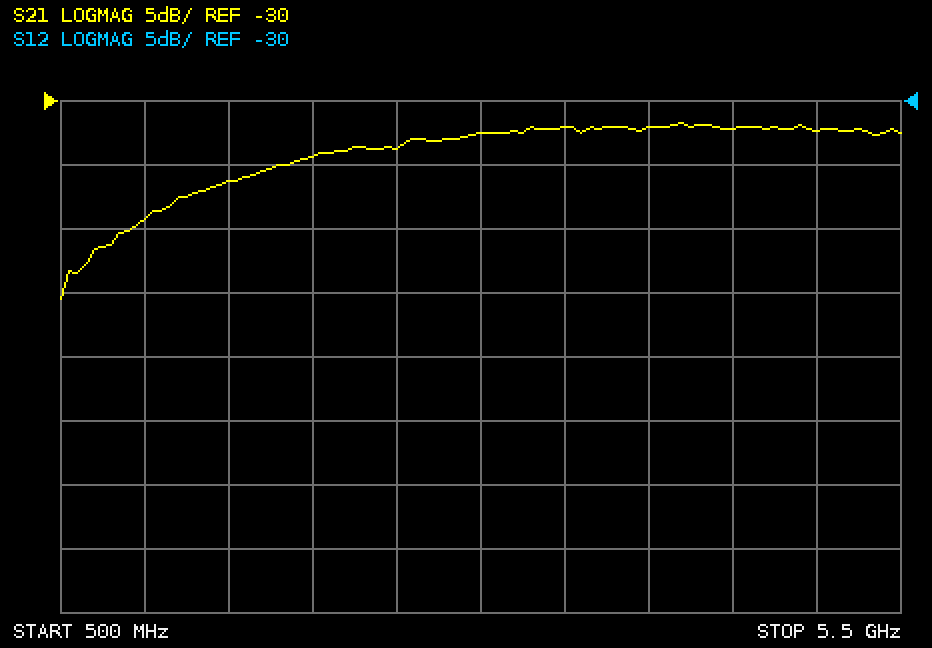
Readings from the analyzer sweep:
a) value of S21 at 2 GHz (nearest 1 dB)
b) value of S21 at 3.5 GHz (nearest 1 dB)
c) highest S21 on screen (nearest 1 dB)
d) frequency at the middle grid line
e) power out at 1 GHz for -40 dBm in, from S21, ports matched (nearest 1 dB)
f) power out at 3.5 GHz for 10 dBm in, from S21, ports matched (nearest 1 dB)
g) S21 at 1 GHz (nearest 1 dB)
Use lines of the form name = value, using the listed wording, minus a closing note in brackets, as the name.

value of S21 at 2 GHz = -34 dB
value of S21 at 3.5 GHz = -32 dB
highest S21 on screen = -32 dB
frequency at the middle grid line = 3 GHz
power out at 1 GHz for -40 dBm in, from S21, ports matched = -79 dBm
power out at 3.5 GHz for 10 dBm in, from S21, ports matched = -22 dBm
S21 at 1 GHz = -39 dB
